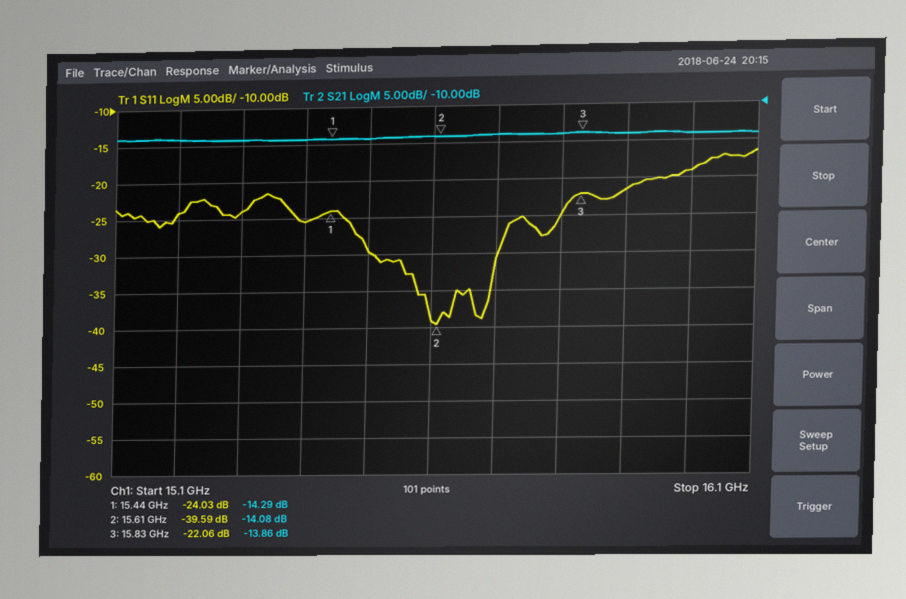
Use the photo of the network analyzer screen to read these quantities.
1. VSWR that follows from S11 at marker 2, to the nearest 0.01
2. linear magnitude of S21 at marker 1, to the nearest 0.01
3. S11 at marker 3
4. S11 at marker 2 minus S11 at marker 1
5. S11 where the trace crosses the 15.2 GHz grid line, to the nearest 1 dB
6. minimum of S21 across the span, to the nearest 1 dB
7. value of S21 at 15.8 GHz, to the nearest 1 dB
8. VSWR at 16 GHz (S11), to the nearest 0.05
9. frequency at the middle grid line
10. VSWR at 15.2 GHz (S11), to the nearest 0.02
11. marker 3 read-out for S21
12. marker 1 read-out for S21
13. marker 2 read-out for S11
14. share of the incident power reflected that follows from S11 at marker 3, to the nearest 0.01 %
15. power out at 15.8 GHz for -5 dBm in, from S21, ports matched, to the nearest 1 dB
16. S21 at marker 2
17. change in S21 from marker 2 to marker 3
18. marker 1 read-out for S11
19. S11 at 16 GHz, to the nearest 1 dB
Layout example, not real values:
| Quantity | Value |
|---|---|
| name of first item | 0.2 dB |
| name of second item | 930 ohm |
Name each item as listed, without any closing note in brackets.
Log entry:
| Quantity | Value |
|---|---|
| VSWR that follows from S11 at marker 2, to the nearest 0.01 | 1.02 |
| linear magnitude of S21 at marker 1, to the nearest 0.01 | 0.19 |
| S11 at marker 3 | -22.06 dB |
| S11 at marker 2 minus S11 at marker 1 | -15.56 dB |
| S11 where the trace crosses the 15.2 GHz grid line, to the nearest 1 dB | -24 dB |
| minimum of S21 across the span, to the nearest 1 dB | -14 dB |
| value of S21 at 15.8 GHz, to the nearest 1 dB | -14 dB |
| VSWR at 16 GHz (S11), to the nearest 0.05 | 1.25 |
| frequency at the middle grid line | 15.6 GHz |
| VSWR at 15.2 GHz (S11), to the nearest 0.02 | 1.14 |
| marker 3 read-out for S21 | -13.86 dB |
| marker 1 read-out for S21 | -14.29 dB |
| marker 2 read-out for S11 | -39.59 dB |
| share of the incident power reflected that follows from S11 at marker 3, to the nearest 0.01 % | 0.62 % |
| power out at 15.8 GHz for -5 dBm in, from S21, ports matched, to the nearest 1 dB | -19 dBm |
| S21 at marker 2 | -14.08 dB |
| change in S21 from marker 2 to marker 3 | 0.22 dB |
| marker 1 read-out for S11 | -24.03 dB |
| S11 at 16 GHz, to the nearest 1 dB | -19 dB |
